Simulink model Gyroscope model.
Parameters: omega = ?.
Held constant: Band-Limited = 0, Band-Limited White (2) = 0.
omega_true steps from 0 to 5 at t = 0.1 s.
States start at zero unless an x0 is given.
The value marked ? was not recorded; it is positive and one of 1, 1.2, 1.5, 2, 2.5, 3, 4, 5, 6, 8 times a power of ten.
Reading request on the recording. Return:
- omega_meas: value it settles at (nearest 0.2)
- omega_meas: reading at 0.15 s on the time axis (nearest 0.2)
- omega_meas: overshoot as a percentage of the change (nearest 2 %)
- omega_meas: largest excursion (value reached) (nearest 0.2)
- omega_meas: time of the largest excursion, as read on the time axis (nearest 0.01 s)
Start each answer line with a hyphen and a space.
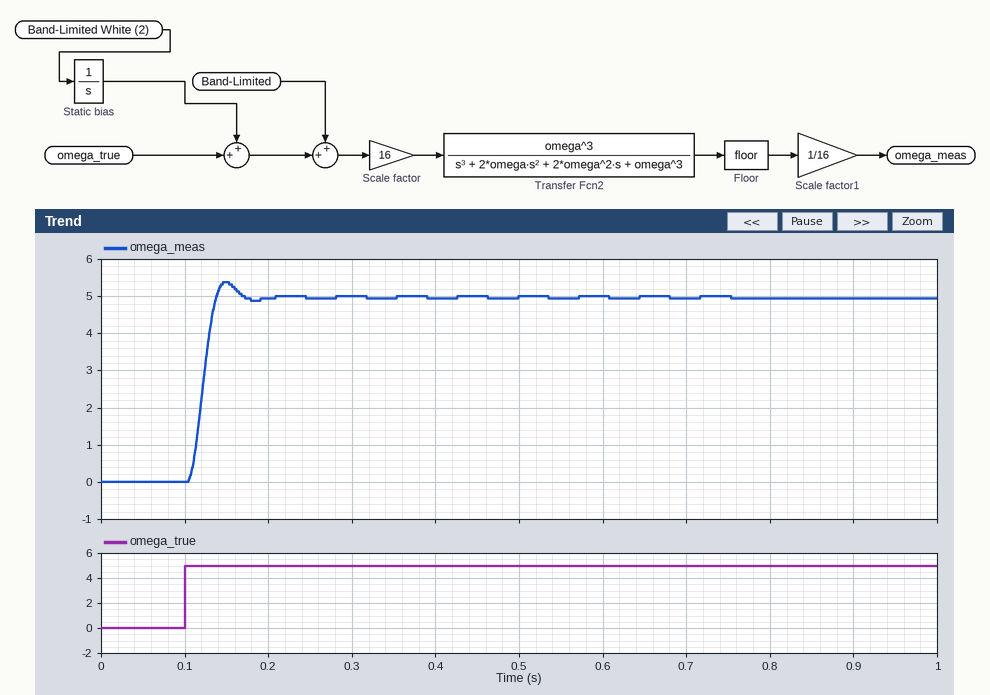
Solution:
- 5.0
- 5.4
- 8 %
- 5.4
- 0.15 s
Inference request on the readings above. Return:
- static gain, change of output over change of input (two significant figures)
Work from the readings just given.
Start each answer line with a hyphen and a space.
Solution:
- 1.0
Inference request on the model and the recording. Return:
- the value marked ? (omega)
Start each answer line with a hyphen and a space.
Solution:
- 100
